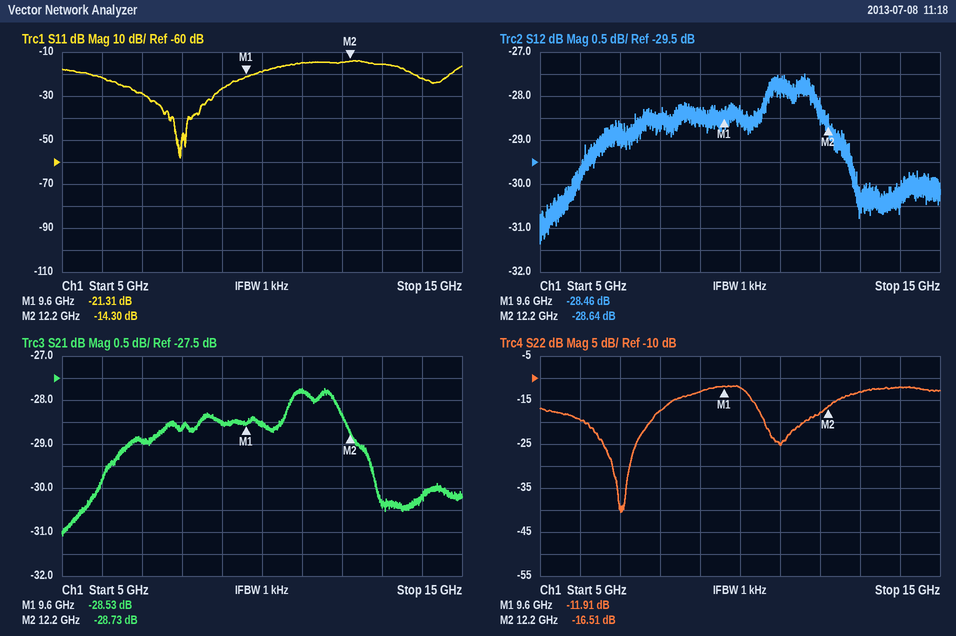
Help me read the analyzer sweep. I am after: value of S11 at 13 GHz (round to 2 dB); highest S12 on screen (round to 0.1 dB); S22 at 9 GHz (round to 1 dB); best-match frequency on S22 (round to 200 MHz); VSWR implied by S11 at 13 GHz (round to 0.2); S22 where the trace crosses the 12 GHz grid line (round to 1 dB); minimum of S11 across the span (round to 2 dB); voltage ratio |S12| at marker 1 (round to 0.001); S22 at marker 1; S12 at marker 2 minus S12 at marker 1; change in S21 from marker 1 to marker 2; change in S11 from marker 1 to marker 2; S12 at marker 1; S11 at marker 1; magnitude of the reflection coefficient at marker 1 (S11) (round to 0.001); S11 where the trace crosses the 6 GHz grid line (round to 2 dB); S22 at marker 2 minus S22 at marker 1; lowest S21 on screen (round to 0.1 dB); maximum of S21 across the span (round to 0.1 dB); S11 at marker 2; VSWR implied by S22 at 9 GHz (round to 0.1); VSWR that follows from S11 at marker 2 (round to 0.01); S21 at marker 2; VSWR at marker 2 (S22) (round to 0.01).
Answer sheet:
-16 dB
-27.5 dB
-13 dB
7.0 GHz
1.4
-18 dB
-58 dB
0.038
-11.91 dB
-0.18 dB
-0.20 dB
7.01 dB
-28.46 dB
-21.31 dB
0.086
-22 dB
-4.60 dB
-31.1 dB
-27.7 dB
-14.30 dB
1.6
1.48
-28.73 dB
1.35
